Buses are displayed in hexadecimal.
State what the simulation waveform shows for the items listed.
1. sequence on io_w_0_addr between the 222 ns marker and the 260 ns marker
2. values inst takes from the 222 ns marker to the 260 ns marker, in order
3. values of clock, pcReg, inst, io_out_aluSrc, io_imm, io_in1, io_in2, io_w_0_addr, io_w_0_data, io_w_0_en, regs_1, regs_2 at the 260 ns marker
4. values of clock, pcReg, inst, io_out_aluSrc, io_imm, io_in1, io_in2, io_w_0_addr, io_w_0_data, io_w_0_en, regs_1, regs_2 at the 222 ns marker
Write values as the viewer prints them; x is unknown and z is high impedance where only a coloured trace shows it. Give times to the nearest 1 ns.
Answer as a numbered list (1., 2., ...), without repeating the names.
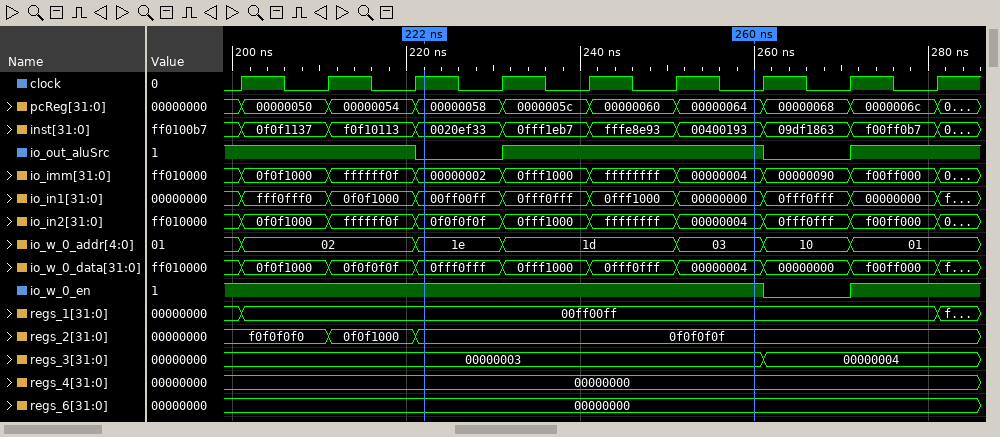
1. 1e, 1d, 03
2. 0020ef33, 0fff1eb7, fffe8e93, 00400193
3. clock=0, pcReg=00000064, inst=00400193, io_out_aluSrc=1, io_imm=00000004, io_in1=00000000, io_in2=00000004, io_w_0_addr=03, io_w_0_data=00000004, io_w_0_en=1, regs_1=00ff00ff, regs_2=0f0f0f0f
4. clock=1, pcReg=00000058, inst=0020ef33, io_out_aluSrc=0, io_imm=00000002, io_in1=00ff00ff, io_in2=0f0f0f0f, io_w_0_addr=1e, io_w_0_data=0fff0fff, io_w_0_en=1, regs_1=00ff00ff, regs_2=0f0f0f0f
